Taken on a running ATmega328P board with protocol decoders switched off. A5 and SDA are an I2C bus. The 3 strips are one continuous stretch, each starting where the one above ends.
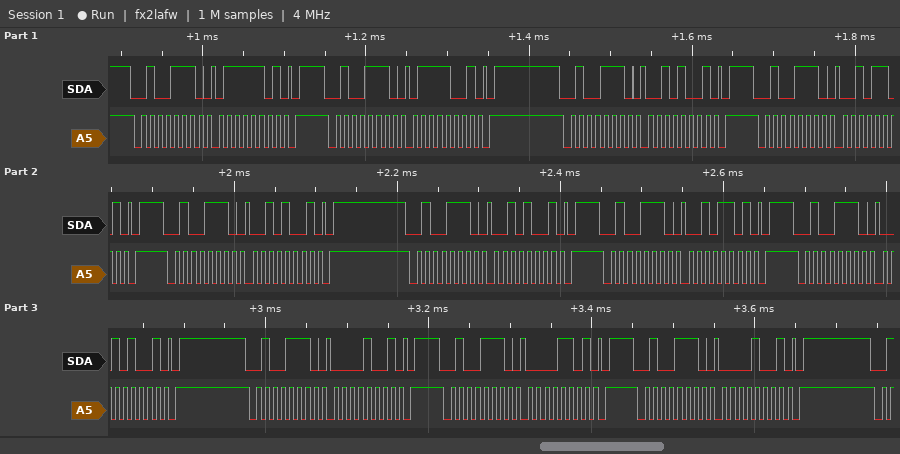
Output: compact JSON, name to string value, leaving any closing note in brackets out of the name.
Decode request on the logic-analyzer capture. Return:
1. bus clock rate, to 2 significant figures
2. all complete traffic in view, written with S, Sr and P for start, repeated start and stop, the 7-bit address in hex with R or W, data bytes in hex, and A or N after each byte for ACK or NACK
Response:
{"bus clock rate, to 2 significant figures": "100 kHz", "all complete traffic in view, written with S, Sr and P for start, repeated start and stop, the 7-bit address in hex with R or W, data bytes in hex, and A or N after each byte for ACK or NACK": "S 27W A 7D A P S 27W A 79 A P S 27W A 29 A P S 27W A 2D A P S 27W A 29 A P S 27W A 29 A P S 27W A 2D A P S 27W A 29 A P S 27W A 09 A P S 27W A 0D A P S 27W A 09 A P"}
